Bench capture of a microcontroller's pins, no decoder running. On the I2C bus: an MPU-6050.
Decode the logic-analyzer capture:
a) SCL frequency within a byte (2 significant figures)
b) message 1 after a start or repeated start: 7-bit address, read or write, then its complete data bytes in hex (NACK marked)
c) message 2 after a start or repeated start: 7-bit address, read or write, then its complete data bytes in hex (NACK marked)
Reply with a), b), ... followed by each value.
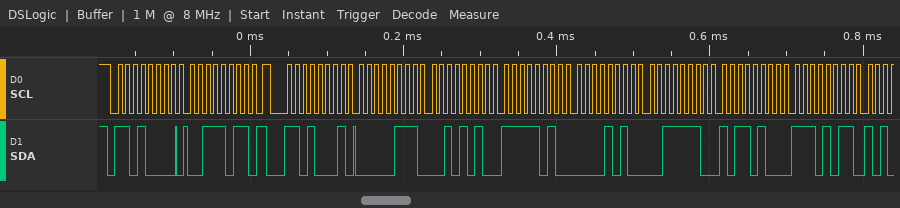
a) 100 kHz
b) 0x68 write: 3B
c) 0x68 read: 07 2A FA 0A 3E B4 EB
